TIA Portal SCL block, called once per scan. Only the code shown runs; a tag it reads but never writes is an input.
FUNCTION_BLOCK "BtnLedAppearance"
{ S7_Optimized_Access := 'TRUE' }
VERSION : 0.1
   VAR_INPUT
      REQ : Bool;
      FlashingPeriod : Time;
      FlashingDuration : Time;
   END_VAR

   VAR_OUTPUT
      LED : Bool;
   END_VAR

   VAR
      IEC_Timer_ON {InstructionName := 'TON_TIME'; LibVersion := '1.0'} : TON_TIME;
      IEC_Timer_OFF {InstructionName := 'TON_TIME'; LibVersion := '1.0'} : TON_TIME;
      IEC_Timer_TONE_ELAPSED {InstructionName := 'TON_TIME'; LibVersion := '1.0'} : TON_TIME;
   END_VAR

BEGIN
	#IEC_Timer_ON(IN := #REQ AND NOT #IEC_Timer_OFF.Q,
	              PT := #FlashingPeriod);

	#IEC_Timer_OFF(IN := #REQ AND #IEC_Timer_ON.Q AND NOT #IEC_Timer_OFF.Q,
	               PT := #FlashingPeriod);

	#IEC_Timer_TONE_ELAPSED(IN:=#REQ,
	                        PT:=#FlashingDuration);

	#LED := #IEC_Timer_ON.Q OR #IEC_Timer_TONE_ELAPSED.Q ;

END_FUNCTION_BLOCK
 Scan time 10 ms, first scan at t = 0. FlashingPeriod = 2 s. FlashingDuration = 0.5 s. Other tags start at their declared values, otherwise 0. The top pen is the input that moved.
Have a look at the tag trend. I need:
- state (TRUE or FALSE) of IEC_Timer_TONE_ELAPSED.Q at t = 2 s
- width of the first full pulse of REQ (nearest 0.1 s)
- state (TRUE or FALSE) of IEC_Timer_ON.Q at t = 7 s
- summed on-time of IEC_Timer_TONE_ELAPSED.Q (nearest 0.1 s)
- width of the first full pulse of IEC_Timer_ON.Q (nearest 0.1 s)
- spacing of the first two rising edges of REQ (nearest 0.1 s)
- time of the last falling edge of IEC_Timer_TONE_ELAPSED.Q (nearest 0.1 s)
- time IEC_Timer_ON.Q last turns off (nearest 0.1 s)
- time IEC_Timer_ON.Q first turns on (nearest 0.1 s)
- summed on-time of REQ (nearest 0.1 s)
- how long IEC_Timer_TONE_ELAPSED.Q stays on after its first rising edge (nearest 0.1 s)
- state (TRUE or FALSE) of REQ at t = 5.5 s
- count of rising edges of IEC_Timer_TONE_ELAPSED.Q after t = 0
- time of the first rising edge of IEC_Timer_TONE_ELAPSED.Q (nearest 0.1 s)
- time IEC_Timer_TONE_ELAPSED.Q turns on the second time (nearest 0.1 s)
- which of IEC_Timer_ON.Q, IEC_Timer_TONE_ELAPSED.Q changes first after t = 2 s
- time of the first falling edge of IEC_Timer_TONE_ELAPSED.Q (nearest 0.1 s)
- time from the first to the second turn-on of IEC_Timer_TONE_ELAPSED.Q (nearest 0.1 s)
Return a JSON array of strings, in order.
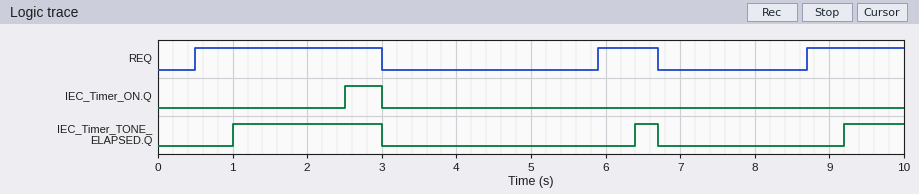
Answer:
["TRUE", "2.5 s", "FALSE", "3.1 s", "0.5 s", "5.4 s", "6.7 s", "3.0 s", "2.5 s", "4.6 s", "2.0 s", "FALSE", "3", "1.0 s", "6.4 s", "IEC_Timer_ON.Q", "3.0 s", "5.4 s"]
